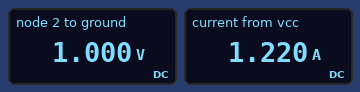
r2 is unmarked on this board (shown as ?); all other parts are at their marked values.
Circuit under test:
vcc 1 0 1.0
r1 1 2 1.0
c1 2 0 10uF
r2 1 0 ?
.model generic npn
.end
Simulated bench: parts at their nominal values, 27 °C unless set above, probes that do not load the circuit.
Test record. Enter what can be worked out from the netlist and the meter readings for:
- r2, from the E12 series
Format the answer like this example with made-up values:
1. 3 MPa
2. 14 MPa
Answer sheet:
1. 0.82 Ω
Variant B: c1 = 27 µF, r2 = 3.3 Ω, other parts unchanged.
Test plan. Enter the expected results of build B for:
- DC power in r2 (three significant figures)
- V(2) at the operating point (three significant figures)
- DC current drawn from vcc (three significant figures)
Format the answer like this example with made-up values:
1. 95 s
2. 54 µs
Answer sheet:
1. 303 mW
2. 1.00 V
3. 303 mA
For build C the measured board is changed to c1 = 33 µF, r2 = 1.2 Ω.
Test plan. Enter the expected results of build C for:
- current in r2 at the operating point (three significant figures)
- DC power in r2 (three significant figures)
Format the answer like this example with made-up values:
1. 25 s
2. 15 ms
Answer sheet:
1. 833 mA
2. 833 mW
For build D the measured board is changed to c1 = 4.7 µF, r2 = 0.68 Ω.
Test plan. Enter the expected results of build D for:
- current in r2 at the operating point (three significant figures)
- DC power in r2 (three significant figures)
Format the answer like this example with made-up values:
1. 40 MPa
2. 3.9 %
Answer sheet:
1. 1.47 A
2. 1.47 W
